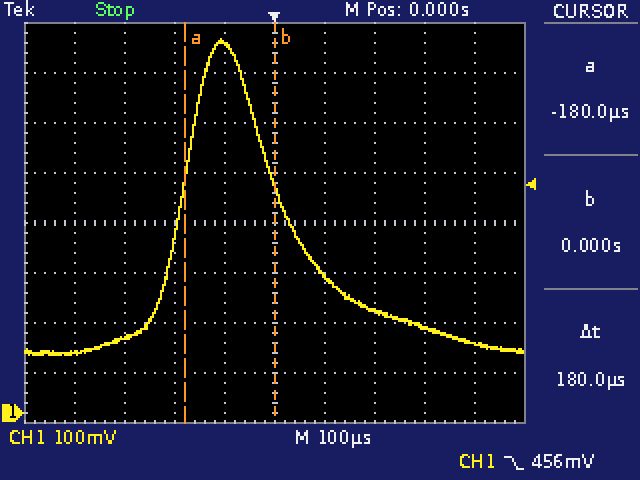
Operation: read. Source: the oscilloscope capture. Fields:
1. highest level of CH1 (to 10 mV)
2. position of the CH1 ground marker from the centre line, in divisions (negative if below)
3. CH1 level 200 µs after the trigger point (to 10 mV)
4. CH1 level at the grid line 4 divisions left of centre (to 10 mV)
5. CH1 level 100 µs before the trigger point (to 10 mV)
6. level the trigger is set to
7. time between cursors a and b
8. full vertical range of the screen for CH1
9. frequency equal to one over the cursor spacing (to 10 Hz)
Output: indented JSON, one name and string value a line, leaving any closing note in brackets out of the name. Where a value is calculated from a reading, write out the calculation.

{
  "highest level of CH1": "750 mV",
  "position of the CH1 ground marker from the centre line, in divisions": "-3.8 div",
  "CH1 level 200 µs after the trigger point": "200 mV",
  "CH1 level at the grid line 4 divisions left of centre": "120 mV",
  "CH1 level 100 µs before the trigger point": "740 mV",
  "level the trigger is set to": "456 mV",
  "time between cursors a and b": "180 µs",
  "full vertical range of the screen for CH1": "800 mV",
  "frequency equal to one over the cursor spacing": "1 / 180 µs ≈ 5.56 kHz"
}
